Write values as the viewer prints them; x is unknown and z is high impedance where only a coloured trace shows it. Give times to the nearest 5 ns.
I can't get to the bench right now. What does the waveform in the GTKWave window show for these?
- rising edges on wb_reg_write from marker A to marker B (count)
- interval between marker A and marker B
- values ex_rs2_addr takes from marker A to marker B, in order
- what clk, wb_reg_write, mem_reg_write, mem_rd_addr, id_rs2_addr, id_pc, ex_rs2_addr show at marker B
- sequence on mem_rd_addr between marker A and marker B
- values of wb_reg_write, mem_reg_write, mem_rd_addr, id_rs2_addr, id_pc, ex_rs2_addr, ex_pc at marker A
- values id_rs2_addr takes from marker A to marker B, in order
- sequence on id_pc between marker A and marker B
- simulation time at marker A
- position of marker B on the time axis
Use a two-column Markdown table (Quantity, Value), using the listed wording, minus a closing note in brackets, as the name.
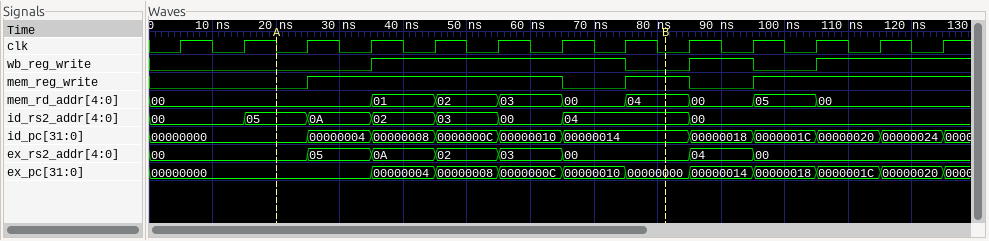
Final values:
| Quantity | Value |
|---|---|
| rising edges on wb_reg_write from marker A to marker B | 1 |
| interval between marker A and marker B | 60 ns |
| values ex_rs2_addr takes from marker A to marker B, in order | 00, 05, 0A, 02, 03, 00 |
| what clk, wb_reg_write, mem_reg_write, mem_rd_addr, id_rs2_addr, id_pc, ex_rs2_addr show at marker B | clk=0, wb_reg_write=0, mem_reg_write=1, mem_rd_addr=04, id_rs2_addr=04, id_pc=00000014, ex_rs2_addr=00 |
| sequence on mem_rd_addr between marker A and marker B | 00, 01, 02, 03, 00, 04 |
| values of wb_reg_write, mem_reg_write, mem_rd_addr, id_rs2_addr, id_pc, ex_rs2_addr, ex_pc at marker A | wb_reg_write=0, mem_reg_write=0, mem_rd_addr=00, id_rs2_addr=05, id_pc=00000000, ex_rs2_addr=00, ex_pc=00000000 |
| values id_rs2_addr takes from marker A to marker B, in order | 05, 0A, 02, 03, 00, 04 |
| sequence on id_pc between marker A and marker B | 00000000, 00000004, 00000008, 0000000C, 00000010, 00000014 |
| simulation time at marker A | 20 ns |
| position of marker B on the time axis | 80 ns |
